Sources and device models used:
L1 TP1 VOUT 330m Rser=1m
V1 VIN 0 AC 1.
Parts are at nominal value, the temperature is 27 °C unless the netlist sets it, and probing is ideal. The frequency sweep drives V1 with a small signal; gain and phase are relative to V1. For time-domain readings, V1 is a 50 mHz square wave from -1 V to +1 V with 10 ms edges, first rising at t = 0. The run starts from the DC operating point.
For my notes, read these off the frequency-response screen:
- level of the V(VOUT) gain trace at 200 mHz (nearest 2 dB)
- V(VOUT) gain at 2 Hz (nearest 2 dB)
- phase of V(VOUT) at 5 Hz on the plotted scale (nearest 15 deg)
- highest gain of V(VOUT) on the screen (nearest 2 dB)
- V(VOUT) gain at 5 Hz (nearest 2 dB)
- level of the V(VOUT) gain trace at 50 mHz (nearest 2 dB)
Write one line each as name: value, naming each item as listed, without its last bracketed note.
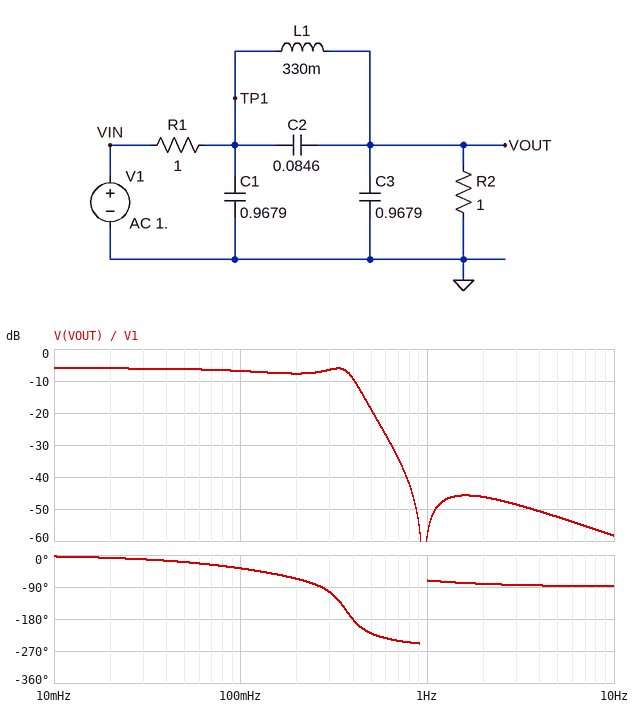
level of the V(VOUT) gain trace at 200 mHz: -8 dB
V(VOUT) gain at 2 Hz: -46 dB
phase of V(VOUT) at 5 Hz on the plotted scale: -90 deg
highest gain of V(VOUT) on the screen: -6 dB
V(VOUT) gain at 5 Hz: -52 dB
level of the V(VOUT) gain trace at 50 mHz: -6 dB
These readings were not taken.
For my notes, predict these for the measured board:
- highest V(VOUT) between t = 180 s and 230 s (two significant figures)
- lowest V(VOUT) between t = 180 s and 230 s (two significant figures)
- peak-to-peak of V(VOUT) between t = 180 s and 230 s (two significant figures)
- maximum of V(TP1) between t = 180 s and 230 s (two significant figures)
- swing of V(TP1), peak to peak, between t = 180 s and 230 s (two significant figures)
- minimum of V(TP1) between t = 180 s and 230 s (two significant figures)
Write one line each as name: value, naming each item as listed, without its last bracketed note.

highest V(VOUT) between t = 180 s and 230 s: 540 mV
lowest V(VOUT) between t = 180 s and 230 s: -540 mV
peak-to-peak of V(VOUT) between t = 180 s and 230 s: 1.1 V
maximum of V(TP1) between t = 180 s and 230 s: 560 mV
swing of V(TP1), peak to peak, between t = 180 s and 230 s: 1.1 V
minimum of V(TP1) between t = 180 s and 230 s: -560 mV
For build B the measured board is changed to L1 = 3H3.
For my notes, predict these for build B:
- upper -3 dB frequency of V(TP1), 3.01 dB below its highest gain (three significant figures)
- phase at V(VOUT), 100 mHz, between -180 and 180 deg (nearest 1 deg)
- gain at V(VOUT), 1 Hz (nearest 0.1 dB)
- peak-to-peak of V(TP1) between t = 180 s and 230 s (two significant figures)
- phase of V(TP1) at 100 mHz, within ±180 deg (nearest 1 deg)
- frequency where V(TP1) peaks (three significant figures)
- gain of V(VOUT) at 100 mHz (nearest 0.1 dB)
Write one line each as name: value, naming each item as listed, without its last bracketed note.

upper -3 dB frequency of V(TP1), 3.01 dB below its highest gain: 227 mHz
phase at V(VOUT), 100 mHz, between -180 and 180 deg: -107 deg
gain at V(VOUT), 1 Hz: -39.2 dB
peak-to-peak of V(TP1) between t = 180 s and 230 s: 1.9 V
phase of V(TP1) at 100 mHz, within ±180 deg: -7 deg
frequency where V(TP1) peaks: 118 mHz
gain of V(VOUT) at 100 mHz: -9.0 dB
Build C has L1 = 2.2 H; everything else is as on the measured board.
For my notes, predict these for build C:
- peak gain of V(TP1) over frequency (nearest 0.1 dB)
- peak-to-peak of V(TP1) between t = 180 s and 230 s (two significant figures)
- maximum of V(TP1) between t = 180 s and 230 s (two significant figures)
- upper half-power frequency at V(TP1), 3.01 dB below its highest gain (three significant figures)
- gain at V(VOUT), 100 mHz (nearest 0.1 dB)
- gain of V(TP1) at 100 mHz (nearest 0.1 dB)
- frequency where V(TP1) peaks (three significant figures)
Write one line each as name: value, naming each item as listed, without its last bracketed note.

peak gain of V(TP1) over frequency: -1.7 dB
peak-to-peak of V(TP1) between t = 180 s and 230 s: 1.7 V
maximum of V(TP1) between t = 180 s and 230 s: 850 mV
upper half-power frequency at V(TP1), 3.01 dB below its highest gain: 254 mHz
gain at V(VOUT), 100 mHz: -6.7 dB
gain of V(TP1) at 100 mHz: -3.2 dB
frequency where V(TP1) peaks: 147 mHz
